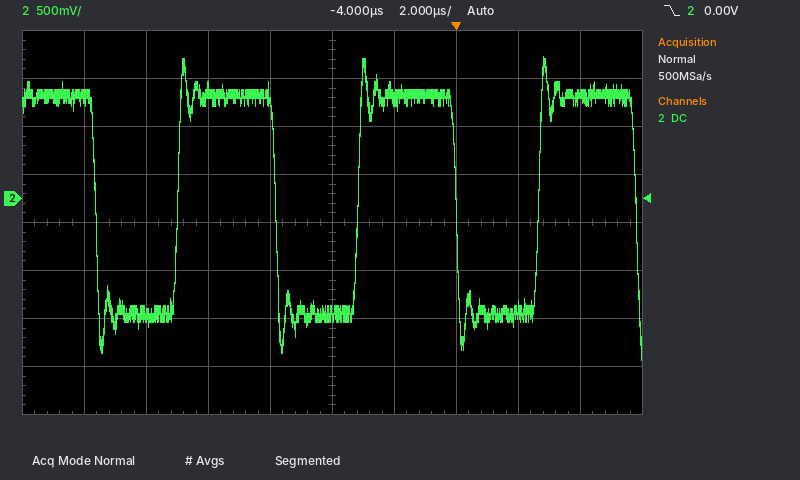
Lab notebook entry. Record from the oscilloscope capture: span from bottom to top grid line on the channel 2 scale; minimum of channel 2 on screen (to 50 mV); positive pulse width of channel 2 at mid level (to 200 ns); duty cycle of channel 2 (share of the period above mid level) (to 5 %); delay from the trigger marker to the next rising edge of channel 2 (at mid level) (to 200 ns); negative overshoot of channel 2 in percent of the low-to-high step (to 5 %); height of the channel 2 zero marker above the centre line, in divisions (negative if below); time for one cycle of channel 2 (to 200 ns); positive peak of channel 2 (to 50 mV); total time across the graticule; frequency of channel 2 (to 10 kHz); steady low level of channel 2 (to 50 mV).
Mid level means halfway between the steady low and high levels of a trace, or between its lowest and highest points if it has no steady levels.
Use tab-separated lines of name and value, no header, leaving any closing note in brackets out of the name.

span from bottom to top grid line on the channel 2 scale	4 V
minimum of channel 2 on screen	-1.70 V
positive pulse width of channel 2 at mid level	3.2 µs
duty cycle of channel 2 (share of the period above mid level)	55 %
delay from the trigger marker to the next rising edge of channel 2 (at mid level)	2.6 µs
negative overshoot of channel 2 in percent of the low-to-high step	20 %
height of the channel 2 zero marker above the centre line, in divisions	+0.5 div
time for one cycle of channel 2	5.8 µs
positive peak of channel 2	1.50 V
total time across the graticule	20 µs
frequency of channel 2	170 kHz
steady low level of channel 2	-1.20 V
